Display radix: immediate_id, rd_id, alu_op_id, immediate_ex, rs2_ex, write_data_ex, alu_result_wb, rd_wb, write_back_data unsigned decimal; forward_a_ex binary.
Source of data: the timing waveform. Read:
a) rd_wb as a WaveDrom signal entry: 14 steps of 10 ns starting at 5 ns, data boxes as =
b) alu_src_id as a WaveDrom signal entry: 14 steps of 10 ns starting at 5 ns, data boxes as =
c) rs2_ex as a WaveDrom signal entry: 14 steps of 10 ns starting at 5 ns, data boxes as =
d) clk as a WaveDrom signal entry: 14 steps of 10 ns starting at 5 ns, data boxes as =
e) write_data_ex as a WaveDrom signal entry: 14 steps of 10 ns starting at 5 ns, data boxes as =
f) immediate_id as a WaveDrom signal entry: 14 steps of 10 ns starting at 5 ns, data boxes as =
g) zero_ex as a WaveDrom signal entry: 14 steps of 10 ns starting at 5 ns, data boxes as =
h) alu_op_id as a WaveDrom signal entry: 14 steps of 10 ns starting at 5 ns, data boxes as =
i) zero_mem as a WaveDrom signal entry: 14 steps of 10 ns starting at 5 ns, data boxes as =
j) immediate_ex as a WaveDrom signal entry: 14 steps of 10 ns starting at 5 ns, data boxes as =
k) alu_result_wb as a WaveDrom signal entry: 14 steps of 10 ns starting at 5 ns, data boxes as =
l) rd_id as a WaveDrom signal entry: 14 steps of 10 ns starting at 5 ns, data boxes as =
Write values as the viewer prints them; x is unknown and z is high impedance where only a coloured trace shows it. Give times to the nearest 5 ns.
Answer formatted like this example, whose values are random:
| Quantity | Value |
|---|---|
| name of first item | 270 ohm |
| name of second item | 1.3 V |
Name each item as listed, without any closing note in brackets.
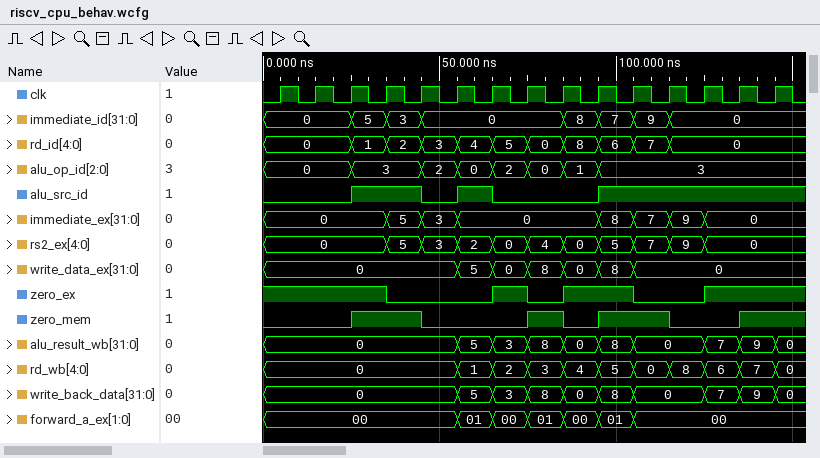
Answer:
| Quantity | Value |
|---|---|
| rd_wb as a WaveDrom signal entry: 14 steps of 10 ns starting at 5 ns, data boxes as = | {name: 'rd_wb', wave: '=....=========', data: '0 1 2 3 4 5 0 8 6 7'} |
| alu_src_id as a WaveDrom signal entry: 14 steps of 10 ns starting at 5 ns, data boxes as = | {name: 'alu_src_id', wave: '0.1.010..1....'} |
| rs2_ex as a WaveDrom signal entry: 14 steps of 10 ns starting at 5 ns, data boxes as = | {name: 'rs2_ex', wave: '=..==========.', data: '0 5 3 2 0 4 0 5 7 9 0'} |
| clk as a WaveDrom signal entry: 14 steps of 10 ns starting at 5 ns, data boxes as = | {name: 'clk', wave: 'p.............'} |
| write_data_ex as a WaveDrom signal entry: 14 steps of 10 ns starting at 5 ns, data boxes as = | {name: 'write_data_ex', wave: '=....======...', data: '0 5 0 8 0 8 0'} |
| immediate_id as a WaveDrom signal entry: 14 steps of 10 ns starting at 5 ns, data boxes as = | {name: 'immediate_id', wave: '=.===...====..', data: '0 5 3 0 8 7 9 0'} |
| zero_ex as a WaveDrom signal entry: 14 steps of 10 ns starting at 5 ns, data boxes as = | {name: 'zero_ex', wave: '1..0..101.0.1.'} |
| alu_op_id as a WaveDrom signal entry: 14 steps of 10 ns starting at 5 ns, data boxes as = | {name: 'alu_op_id', wave: '=.=.======....', data: '0 3 2 0 2 0 1 3'} |
| zero_mem as a WaveDrom signal entry: 14 steps of 10 ns starting at 5 ns, data boxes as = | {name: 'zero_mem', wave: '0.1.0..101.0.1'} |
| immediate_ex as a WaveDrom signal entry: 14 steps of 10 ns starting at 5 ns, data boxes as = | {name: 'immediate_ex', wave: '=..===...====.', data: '0 5 3 0 8 7 9 0'} |
| alu_result_wb as a WaveDrom signal entry: 14 steps of 10 ns starting at 5 ns, data boxes as = | {name: 'alu_result_wb', wave: '=....======.==', data: '0 5 3 8 0 8 0 7 9'} |
| rd_id as a WaveDrom signal entry: 14 steps of 10 ns starting at 5 ns, data boxes as = | {name: 'rd_id', wave: '=.==========..', data: '0 1 2 3 4 5 0 8 6 7 0'} |
